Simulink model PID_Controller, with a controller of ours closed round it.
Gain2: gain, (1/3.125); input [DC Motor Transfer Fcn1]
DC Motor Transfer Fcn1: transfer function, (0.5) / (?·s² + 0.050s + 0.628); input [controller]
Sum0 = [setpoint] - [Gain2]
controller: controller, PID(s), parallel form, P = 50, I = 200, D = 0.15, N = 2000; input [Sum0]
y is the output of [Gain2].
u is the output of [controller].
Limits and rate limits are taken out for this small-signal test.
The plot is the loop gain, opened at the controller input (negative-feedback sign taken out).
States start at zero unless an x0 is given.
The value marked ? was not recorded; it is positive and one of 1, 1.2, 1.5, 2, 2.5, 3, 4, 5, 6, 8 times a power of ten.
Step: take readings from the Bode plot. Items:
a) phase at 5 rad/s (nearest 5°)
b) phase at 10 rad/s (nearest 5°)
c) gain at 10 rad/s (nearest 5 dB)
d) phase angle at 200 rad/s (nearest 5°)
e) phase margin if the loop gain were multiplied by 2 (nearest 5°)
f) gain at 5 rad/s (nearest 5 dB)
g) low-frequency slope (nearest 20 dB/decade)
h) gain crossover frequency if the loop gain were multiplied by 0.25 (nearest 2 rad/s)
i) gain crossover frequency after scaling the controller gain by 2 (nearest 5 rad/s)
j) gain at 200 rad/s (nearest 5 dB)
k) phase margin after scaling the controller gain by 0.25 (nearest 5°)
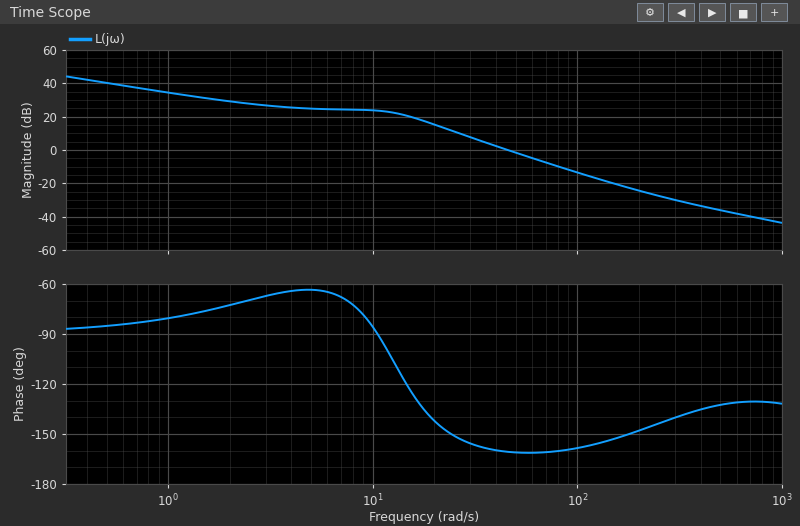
-65°
-85°
25 dB
-150°
20°
25 dB
-20 dB/decade
24 rad/s
65 rad/s
-25 dB
30°
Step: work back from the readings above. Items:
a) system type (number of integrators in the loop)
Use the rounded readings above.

1
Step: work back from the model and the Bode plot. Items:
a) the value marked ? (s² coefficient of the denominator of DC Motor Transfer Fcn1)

0.004
